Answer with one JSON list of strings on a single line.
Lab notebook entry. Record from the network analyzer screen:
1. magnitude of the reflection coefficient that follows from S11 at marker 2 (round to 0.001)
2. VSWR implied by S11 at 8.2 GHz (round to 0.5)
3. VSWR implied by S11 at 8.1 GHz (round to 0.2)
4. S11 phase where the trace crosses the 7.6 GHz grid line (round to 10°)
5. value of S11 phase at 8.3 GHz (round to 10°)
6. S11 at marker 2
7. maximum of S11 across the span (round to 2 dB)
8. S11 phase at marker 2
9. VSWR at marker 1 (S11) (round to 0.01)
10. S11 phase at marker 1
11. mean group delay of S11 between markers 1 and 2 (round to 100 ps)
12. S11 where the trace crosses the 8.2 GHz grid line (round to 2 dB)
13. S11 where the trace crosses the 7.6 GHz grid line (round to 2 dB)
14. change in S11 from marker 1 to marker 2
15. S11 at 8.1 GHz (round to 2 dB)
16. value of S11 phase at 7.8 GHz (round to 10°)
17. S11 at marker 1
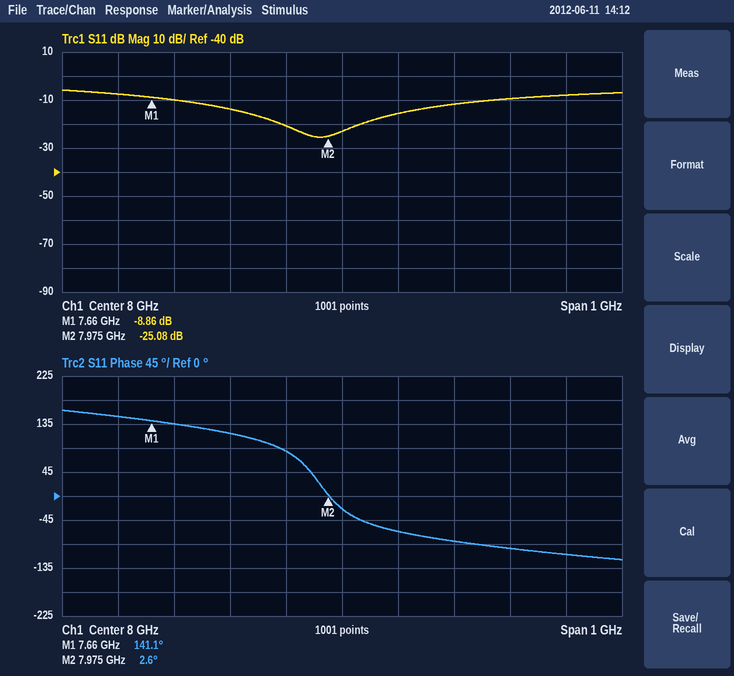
["0.056", "1.5", "1.4", "150°", "-100°", "-25.08 dB", "-6 dB", "2.6°", "2.13", "141.1°", "1.2 ns", "-12 dB", "-8 dB", "-16.22 dB", "-16 dB", "120°", "-8.86 dB"]
